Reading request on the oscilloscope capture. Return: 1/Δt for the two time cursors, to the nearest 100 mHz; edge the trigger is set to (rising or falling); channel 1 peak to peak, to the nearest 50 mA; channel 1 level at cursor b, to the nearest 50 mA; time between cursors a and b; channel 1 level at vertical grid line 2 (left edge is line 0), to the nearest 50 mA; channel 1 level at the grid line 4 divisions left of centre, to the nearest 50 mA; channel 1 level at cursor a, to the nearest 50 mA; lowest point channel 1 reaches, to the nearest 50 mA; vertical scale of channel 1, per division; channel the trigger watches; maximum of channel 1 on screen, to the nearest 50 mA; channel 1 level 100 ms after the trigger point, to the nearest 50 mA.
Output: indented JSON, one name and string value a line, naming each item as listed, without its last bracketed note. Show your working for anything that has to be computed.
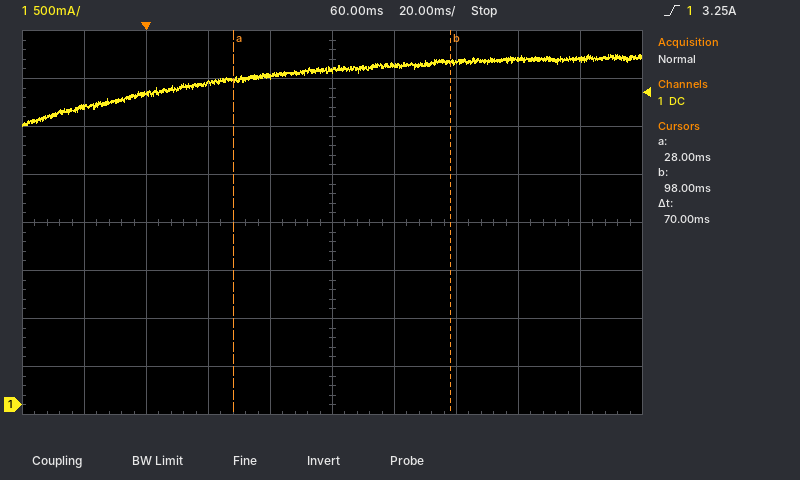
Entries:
{
  "1/Δt for the two time cursors, to the nearest 100 mHz": "1 / 70 ms ≈ 14.3 Hz",
  "edge the trigger is set to": "rising",
  "channel 1 peak to peak, to the nearest 50 mA": "3.65 A − (2.90 A) = 750 mA",
  "channel 1 level at cursor b, to the nearest 50 mA": "3.55 A",
  "time between cursors a and b": "70 ms",
  "channel 1 level at vertical grid line 2 (left edge is line 0), to the nearest 50 mA": "3.25 A",
  "channel 1 level at the grid line 4 divisions left of centre, to the nearest 50 mA": "3.10 A",
  "channel 1 level at cursor a, to the nearest 50 mA": "3.40 A",
  "lowest point channel 1 reaches, to the nearest 50 mA": "2.90 A",
  "vertical scale of channel 1, per division": "500 mA",
  "channel the trigger watches": "channel 1",
  "maximum of channel 1 on screen, to the nearest 50 mA": "3.65 A",
  "channel 1 level 100 ms after the trigger point, to the nearest 50 mA": "3.55 A"
}
